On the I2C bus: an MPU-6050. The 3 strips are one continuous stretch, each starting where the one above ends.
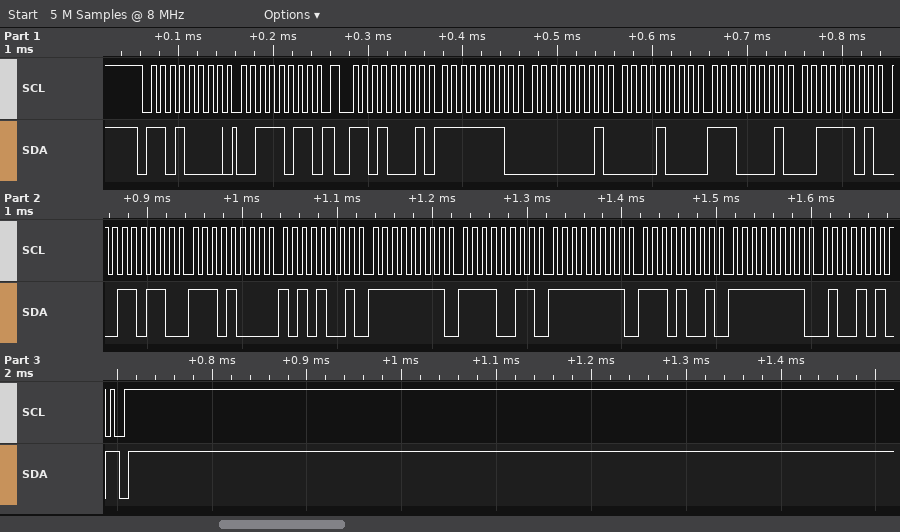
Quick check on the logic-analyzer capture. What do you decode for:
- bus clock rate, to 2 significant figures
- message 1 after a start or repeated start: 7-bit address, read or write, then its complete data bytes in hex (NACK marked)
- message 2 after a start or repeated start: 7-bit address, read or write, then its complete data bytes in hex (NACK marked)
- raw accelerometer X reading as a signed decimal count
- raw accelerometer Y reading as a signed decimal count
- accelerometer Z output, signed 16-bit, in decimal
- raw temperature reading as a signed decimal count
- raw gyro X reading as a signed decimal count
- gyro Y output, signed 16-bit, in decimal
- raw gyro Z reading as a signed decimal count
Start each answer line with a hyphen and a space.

- 100 kHz
- 0x68 write: 3B
- 0x68 read: FE 01 08 E1 3D 36 E8 A9 FF F3 FF E9 FF 4A NACK
- -511
- 2273
- 15670
- -5975
- -13
- -23
- -182
